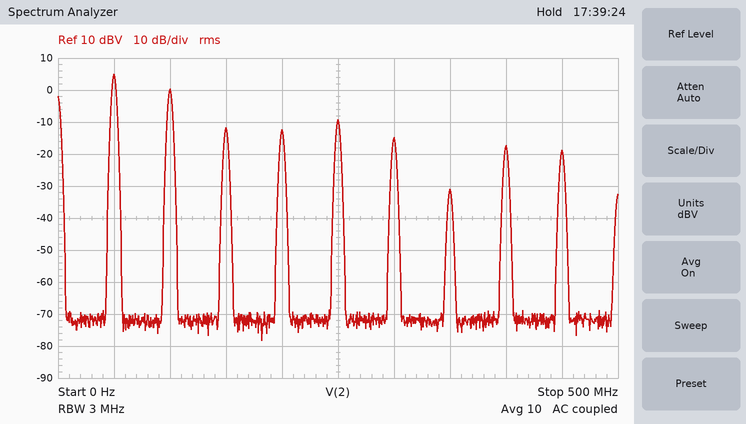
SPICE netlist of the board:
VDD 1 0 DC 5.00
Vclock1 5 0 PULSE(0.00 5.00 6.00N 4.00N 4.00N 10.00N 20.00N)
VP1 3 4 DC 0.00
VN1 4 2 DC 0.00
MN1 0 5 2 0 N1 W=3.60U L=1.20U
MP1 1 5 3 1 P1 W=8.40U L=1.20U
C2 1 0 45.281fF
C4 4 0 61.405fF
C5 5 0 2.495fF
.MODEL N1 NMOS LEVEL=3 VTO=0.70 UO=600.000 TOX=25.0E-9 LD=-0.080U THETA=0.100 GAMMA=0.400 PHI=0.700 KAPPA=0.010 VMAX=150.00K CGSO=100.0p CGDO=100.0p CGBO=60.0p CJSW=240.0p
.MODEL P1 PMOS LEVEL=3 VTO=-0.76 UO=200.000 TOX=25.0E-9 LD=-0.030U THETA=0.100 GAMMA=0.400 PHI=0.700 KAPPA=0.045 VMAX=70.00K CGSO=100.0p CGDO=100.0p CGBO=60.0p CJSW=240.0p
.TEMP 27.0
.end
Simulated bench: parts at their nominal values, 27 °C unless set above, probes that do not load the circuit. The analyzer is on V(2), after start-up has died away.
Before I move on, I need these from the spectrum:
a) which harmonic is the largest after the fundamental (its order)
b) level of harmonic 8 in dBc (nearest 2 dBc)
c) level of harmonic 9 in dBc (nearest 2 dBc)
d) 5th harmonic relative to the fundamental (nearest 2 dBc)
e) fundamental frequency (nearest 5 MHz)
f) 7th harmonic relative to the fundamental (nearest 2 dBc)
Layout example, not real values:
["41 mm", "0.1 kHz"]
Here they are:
["2", "-22 dBc", "-24 dBc", "-14 dBc", "50 MHz", "-36 dBc"]
